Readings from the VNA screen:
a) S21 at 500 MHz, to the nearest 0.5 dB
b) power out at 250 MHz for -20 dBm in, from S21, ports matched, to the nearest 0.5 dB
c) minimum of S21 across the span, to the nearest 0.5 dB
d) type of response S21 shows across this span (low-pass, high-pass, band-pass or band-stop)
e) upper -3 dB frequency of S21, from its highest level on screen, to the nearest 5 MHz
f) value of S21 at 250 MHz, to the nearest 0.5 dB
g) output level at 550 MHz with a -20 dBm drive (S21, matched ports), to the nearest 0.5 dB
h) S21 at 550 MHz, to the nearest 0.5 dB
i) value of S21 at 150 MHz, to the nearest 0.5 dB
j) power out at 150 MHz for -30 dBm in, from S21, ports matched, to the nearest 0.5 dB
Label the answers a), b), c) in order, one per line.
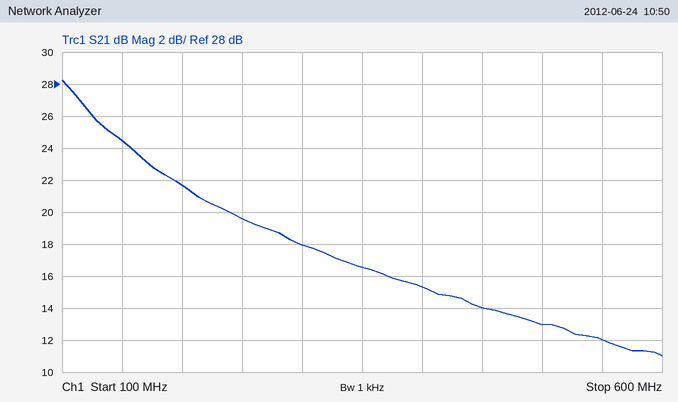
a) 13.0 dB
b) -0.5 dBm
c) 11.0 dB
d) low-pass
e) 135 MHz
f) 19.5 dB
g) -8.0 dBm
h) 12.0 dB
i) 24.5 dB
j) -5.5 dBm
